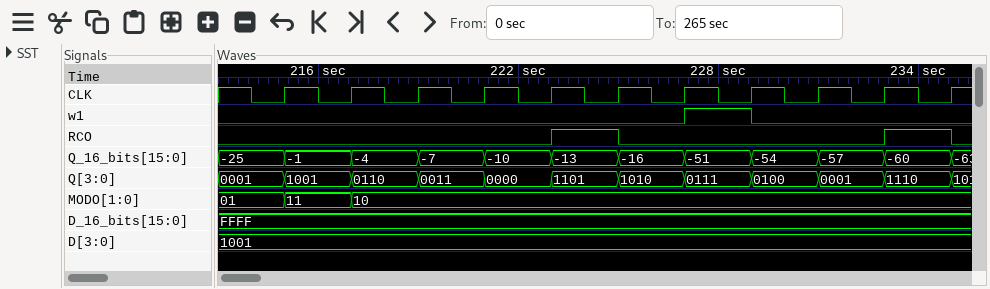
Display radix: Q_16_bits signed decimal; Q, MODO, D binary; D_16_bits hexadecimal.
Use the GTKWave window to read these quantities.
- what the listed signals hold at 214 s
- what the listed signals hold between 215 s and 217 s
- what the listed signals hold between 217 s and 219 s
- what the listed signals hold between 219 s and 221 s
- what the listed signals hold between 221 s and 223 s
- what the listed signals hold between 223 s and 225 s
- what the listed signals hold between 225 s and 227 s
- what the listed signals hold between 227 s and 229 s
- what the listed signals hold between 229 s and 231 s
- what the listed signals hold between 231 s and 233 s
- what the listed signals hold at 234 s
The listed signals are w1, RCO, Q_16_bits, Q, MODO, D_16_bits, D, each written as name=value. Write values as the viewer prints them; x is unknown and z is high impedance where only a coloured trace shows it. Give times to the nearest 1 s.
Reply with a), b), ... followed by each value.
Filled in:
a) w1=0, RCO=0, Q_16_bits=-25, Q=0001, MODO=01, D_16_bits=FFFF, D=1001
b) w1=0, RCO=0, Q_16_bits=-1, Q=1001, MODO=11, D_16_bits=FFFF, D=1001
c) w1=0, RCO=0, Q_16_bits=-4, Q=0110, MODO=10, D_16_bits=FFFF, D=1001
d) w1=0, RCO=0, Q_16_bits=-7, Q=0011, MODO=10, D_16_bits=FFFF, D=1001
e) w1=0, RCO=0, Q_16_bits=-10, Q=0000, MODO=10, D_16_bits=FFFF, D=1001
f) w1=0, RCO=1, Q_16_bits=-13, Q=1101, MODO=10, D_16_bits=FFFF, D=1001
g) w1=0, RCO=0, Q_16_bits=-16, Q=1010, MODO=10, D_16_bits=FFFF, D=1001
h) w1=1, RCO=0, Q_16_bits=-51, Q=0111, MODO=10, D_16_bits=FFFF, D=1001
i) w1=0, RCO=0, Q_16_bits=-54, Q=0100, MODO=10, D_16_bits=FFFF, D=1001
j) w1=0, RCO=0, Q_16_bits=-57, Q=0001, MODO=10, D_16_bits=FFFF, D=1001
k) w1=0, RCO=1, Q_16_bits=-60, Q=1110, MODO=10, D_16_bits=FFFF, D=1001
